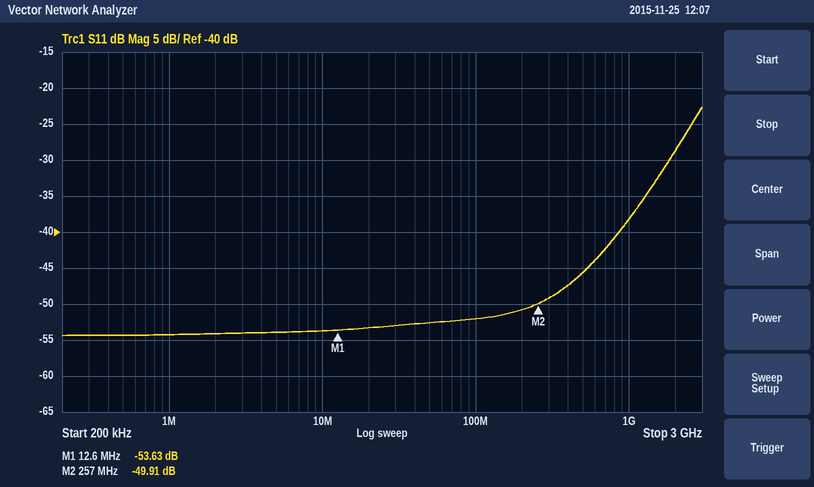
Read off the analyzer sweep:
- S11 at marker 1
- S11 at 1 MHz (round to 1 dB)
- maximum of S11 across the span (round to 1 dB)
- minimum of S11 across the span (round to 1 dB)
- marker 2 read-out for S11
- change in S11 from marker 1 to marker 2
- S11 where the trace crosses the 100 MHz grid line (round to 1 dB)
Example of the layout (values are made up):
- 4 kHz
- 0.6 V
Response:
- -53.63 dB
- -54 dB
- -23 dB
- -54 dB
- -49.91 dB
- 3.72 dB
- -52 dB
